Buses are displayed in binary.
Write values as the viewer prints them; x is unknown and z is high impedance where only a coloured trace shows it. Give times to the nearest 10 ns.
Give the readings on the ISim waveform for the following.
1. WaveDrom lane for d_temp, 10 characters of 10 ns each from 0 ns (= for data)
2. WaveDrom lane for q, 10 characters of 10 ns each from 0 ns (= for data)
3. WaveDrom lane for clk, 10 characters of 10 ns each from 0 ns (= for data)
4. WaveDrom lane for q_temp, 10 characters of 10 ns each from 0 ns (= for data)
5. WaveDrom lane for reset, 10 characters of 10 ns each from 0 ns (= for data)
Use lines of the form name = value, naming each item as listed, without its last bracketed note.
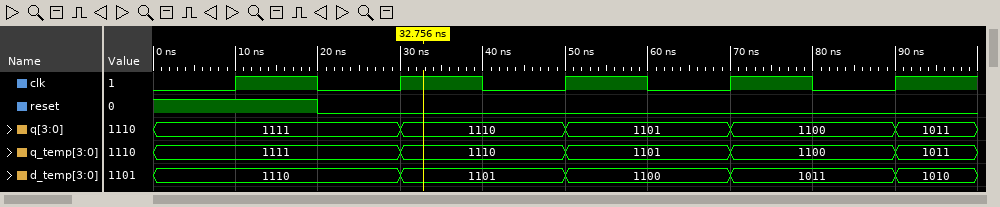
WaveDrom lane for d_temp, 10 characters of 10 ns each from 0 ns = {name: 'd_temp', wave: '=..=.=.=.=', data: '1110 1101 1100 1011 1010'}
WaveDrom lane for q, 10 characters of 10 ns each from 0 ns = {name: 'q', wave: '=..=.=.=.=', data: '1111 1110 1101 1100 1011'}
WaveDrom lane for clk, 10 characters of 10 ns each from 0 ns = {name: 'clk', wave: '0101010101'}
WaveDrom lane for q_temp, 10 characters of 10 ns each from 0 ns = {name: 'q_temp', wave: '=..=.=.=.=', data: '1111 1110 1101 1100 1011'}
WaveDrom lane for reset, 10 characters of 10 ns each from 0 ns = {name: 'reset', wave: '1.0.......'}
